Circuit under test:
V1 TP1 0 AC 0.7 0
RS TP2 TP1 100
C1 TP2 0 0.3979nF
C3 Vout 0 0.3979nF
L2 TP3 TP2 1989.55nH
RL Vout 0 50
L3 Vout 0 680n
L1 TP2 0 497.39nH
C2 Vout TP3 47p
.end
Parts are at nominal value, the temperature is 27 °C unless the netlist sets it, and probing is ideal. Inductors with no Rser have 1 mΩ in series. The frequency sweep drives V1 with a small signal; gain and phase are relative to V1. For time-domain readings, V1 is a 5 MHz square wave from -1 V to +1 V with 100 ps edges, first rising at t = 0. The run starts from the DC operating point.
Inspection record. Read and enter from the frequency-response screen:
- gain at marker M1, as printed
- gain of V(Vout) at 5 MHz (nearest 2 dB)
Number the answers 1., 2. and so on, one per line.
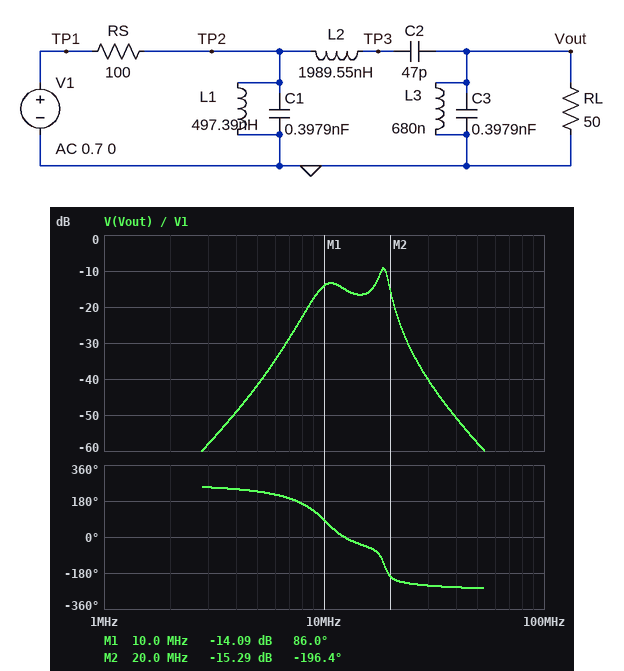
1. -14.09 dB
2. -42 dB
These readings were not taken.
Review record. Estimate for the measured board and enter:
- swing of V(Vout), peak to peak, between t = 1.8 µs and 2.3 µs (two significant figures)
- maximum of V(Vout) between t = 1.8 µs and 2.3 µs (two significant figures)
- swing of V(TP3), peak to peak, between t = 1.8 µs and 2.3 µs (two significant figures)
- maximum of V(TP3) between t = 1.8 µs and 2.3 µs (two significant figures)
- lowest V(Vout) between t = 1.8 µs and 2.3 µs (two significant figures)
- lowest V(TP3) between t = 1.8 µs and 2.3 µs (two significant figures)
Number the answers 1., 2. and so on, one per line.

1. 150 mV
2. 74 mV
3. 1.4 V
4. 700 mV
5. -74 mV
6. -700 mV
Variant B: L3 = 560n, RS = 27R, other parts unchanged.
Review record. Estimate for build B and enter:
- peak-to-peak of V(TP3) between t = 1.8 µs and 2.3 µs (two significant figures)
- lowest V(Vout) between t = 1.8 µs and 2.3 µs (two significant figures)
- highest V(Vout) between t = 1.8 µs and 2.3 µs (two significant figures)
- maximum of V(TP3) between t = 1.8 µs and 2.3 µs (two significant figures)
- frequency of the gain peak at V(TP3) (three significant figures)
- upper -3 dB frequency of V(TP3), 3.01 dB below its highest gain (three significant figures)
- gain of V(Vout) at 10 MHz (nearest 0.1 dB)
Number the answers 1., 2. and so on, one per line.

1. 4.0 V
2. -200 mV
3. 200 mV
4. 2.0 V
5. 18.0 MHz
6. 19.3 MHz
7. -12.9 dB
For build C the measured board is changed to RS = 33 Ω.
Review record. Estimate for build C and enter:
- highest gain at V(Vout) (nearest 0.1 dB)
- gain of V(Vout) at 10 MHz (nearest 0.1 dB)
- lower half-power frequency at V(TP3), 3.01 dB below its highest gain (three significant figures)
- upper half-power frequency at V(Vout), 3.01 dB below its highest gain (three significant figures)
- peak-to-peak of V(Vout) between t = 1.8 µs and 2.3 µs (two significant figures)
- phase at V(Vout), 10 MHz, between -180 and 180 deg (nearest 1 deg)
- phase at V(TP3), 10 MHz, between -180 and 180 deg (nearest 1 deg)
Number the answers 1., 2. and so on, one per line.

1. -4.3 dB
2. -13.3 dB
3. 16.6 MHz
4. 19.3 MHz
5. 350 mV
6. 77 deg
7. 0 deg
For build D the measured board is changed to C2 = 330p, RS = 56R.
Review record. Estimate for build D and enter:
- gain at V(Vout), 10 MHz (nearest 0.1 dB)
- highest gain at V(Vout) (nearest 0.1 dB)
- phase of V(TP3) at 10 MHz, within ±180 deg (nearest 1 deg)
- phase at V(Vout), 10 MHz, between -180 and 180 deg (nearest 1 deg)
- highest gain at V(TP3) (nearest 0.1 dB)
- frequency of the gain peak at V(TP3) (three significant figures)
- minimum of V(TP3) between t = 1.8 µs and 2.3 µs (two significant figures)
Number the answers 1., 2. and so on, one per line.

1. -9.2 dB
2. -7.1 dB
3. -68 deg
4. -26 deg
5. 3.3 dB
6. 4.78 MHz
7. -1.7 V
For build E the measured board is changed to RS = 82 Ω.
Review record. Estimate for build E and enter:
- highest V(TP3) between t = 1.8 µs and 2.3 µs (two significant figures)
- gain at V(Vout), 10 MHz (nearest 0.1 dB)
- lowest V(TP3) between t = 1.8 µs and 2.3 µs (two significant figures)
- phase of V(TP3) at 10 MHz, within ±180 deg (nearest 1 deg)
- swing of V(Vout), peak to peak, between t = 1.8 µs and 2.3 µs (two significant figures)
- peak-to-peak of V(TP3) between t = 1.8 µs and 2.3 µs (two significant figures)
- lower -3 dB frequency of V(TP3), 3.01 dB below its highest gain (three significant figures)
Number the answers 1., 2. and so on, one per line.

1. 840 mV
2. -13.9 dB
3. -840 mV
4. 7 deg
5. 180 mV
6. 1.7 V
7. 17.5 MHz
